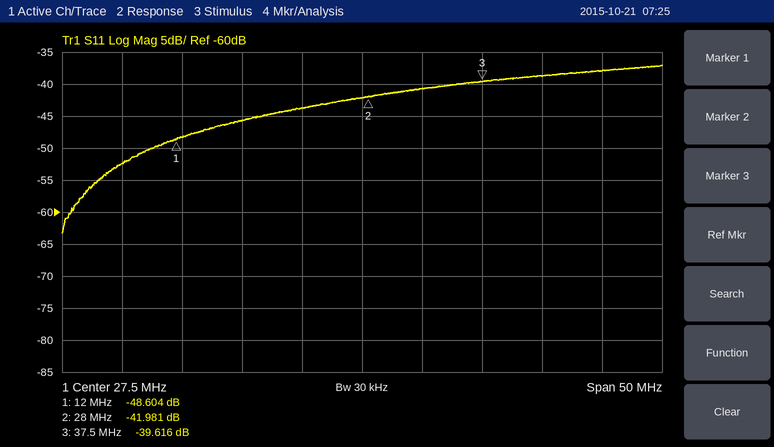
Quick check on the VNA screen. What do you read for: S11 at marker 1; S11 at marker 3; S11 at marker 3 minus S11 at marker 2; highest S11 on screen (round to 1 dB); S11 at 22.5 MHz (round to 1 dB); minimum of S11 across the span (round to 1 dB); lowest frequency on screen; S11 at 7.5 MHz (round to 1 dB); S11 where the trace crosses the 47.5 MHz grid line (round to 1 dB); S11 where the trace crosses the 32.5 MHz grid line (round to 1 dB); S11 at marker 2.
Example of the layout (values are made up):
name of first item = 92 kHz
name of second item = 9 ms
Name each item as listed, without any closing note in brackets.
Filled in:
S11 at marker 1 = -48.604 dB
S11 at marker 3 = -39.616 dB
S11 at marker 3 minus S11 at marker 2 = 2.365 dB
highest S11 on screen = -37 dB
S11 at 22.5 MHz = -44 dB
minimum of S11 across the span = -63 dB
lowest frequency on screen = 2.5 MHz
S11 at 7.5 MHz = -52 dB
S11 where the trace crosses the 47.5 MHz grid line = -38 dB
S11 where the trace crosses the 32.5 MHz grid line = -41 dB
S11 at marker 2 = -41.981 dB
